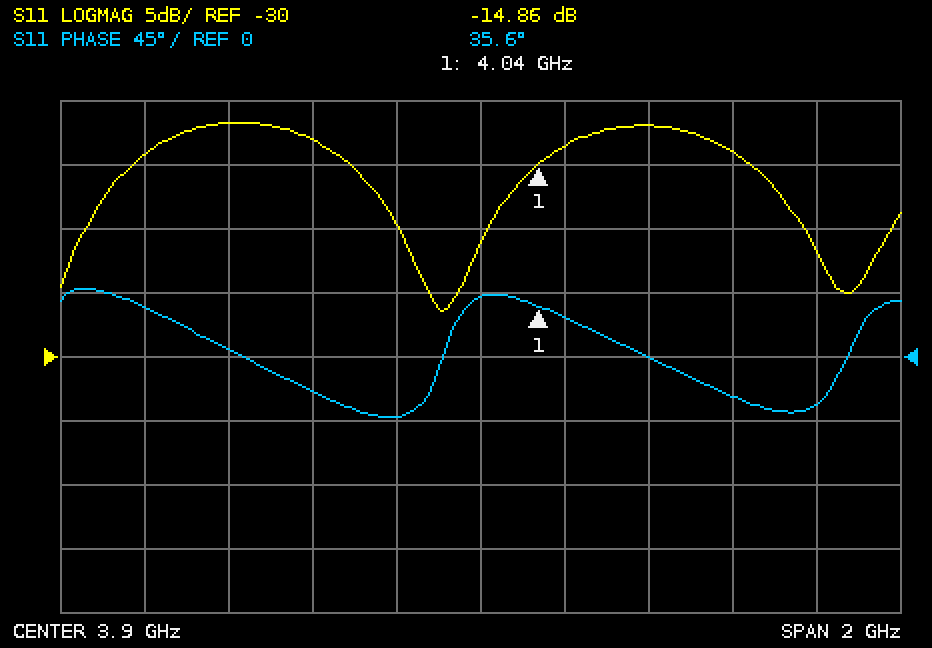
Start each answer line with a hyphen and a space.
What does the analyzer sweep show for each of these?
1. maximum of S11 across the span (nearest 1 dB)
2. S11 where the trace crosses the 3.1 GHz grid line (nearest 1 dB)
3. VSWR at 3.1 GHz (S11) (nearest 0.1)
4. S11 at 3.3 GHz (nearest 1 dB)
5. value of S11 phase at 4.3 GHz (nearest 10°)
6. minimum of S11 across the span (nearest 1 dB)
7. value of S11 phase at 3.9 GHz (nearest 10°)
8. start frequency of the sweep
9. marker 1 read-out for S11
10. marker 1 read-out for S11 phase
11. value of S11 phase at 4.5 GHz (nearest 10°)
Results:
- -12 dB
- -14 dB
- 1.5
- -12 dB
- 0°
- -26 dB
- 40°
- 2.9 GHz
- -14.86 dB
- 35.6°
- -30°
